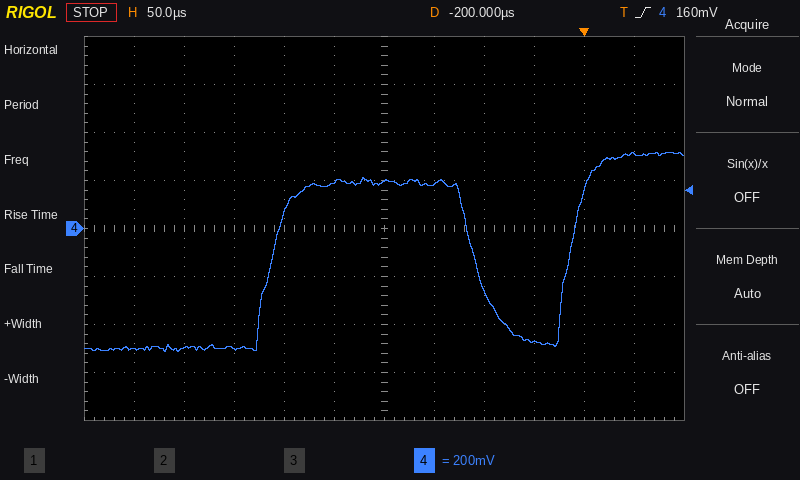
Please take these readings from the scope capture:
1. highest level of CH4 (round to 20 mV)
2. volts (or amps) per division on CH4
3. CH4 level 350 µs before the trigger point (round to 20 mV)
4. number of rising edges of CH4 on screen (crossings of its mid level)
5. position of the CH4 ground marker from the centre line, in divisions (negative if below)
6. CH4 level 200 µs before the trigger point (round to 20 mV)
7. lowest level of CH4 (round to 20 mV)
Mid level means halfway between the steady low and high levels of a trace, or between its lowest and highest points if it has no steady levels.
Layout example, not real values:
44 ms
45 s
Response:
320 mV
200 mV
-500 mV
2
0.0 div
200 mV
-520 mV
